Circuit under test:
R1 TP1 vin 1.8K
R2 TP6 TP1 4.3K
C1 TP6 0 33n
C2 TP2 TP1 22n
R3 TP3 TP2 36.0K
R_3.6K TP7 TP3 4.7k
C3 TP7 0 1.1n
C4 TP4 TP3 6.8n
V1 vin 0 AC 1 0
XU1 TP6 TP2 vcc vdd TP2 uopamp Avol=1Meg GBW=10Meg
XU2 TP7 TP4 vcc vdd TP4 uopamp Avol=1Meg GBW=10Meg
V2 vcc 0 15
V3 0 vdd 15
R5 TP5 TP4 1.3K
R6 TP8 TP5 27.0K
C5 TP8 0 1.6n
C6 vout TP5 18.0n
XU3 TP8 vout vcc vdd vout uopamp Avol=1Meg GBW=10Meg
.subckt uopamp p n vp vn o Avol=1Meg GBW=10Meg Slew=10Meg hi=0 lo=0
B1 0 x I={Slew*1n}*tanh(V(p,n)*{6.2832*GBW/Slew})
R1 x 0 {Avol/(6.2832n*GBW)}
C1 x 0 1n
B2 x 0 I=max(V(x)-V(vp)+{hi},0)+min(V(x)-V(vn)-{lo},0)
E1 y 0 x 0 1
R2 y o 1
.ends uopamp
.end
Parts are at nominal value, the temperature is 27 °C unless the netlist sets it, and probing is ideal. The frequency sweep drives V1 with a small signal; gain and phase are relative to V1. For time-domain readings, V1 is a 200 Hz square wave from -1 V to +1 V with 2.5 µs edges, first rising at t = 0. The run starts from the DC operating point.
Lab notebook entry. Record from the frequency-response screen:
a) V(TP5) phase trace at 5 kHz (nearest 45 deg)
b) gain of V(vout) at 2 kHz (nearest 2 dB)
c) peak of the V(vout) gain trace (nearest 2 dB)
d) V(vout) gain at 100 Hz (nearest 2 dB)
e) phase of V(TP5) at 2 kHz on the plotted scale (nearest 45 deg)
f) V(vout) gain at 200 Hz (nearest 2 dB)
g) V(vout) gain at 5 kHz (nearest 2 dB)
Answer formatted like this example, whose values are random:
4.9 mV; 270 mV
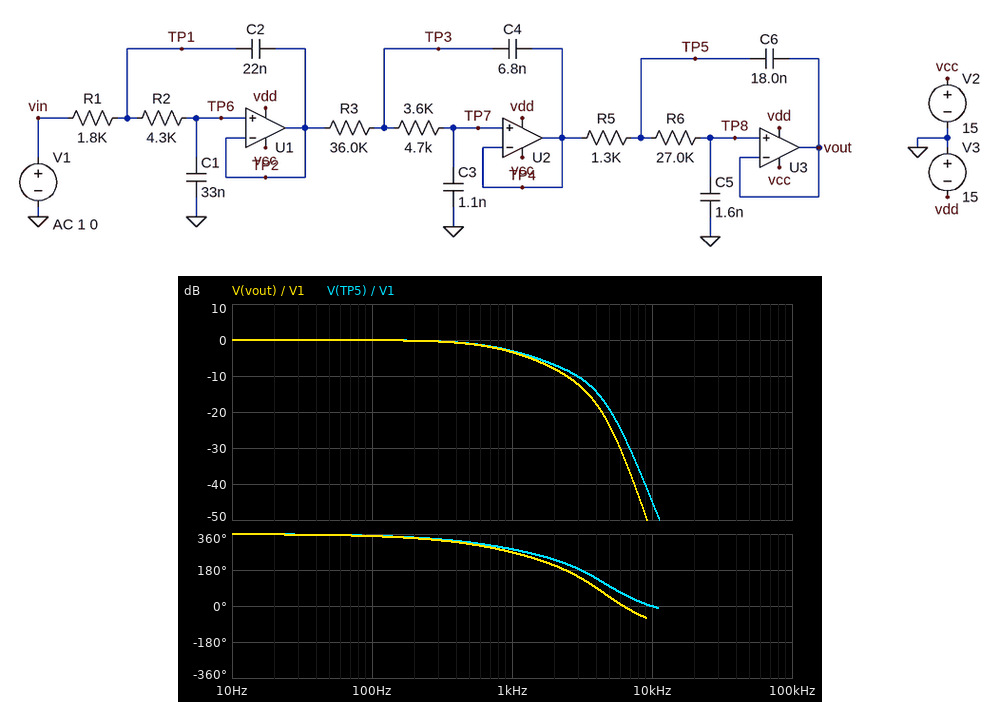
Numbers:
90 deg; -8 dB; 0 dB; 0 dB; 225 deg; 0 dB; -24 dB
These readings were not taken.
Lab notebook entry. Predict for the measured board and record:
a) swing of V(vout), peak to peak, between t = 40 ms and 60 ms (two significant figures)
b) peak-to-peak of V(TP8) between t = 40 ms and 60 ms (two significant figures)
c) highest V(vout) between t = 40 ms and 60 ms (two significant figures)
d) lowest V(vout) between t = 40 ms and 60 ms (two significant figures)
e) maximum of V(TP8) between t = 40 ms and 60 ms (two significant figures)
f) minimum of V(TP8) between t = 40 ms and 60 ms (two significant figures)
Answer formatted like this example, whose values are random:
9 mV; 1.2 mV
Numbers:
2.0 V; 2.0 V; 1.0 V; -1.0 V; 1.0 V; -1.0 V
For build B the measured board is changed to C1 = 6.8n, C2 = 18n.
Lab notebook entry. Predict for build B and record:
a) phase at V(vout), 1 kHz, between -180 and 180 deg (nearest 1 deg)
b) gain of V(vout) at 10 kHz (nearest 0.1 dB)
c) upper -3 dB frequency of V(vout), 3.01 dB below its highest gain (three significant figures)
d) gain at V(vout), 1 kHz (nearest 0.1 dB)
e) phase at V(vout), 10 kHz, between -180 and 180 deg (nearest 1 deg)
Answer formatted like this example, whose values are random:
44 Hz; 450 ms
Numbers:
-48 deg; -37.7 dB; 3.78 kHz; 0.1 dB; -58 deg
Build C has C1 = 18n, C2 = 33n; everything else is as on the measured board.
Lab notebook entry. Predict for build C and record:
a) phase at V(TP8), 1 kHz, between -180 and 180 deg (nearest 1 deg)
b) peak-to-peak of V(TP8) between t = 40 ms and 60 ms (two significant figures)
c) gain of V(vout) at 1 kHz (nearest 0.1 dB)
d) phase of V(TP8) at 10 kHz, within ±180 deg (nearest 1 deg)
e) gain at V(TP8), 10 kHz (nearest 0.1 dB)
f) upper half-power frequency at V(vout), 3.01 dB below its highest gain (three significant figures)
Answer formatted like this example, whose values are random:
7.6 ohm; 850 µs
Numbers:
-73 deg; 2.1 V; -0.5 dB; -80 deg; -51.5 dB; 2.03 kHz
